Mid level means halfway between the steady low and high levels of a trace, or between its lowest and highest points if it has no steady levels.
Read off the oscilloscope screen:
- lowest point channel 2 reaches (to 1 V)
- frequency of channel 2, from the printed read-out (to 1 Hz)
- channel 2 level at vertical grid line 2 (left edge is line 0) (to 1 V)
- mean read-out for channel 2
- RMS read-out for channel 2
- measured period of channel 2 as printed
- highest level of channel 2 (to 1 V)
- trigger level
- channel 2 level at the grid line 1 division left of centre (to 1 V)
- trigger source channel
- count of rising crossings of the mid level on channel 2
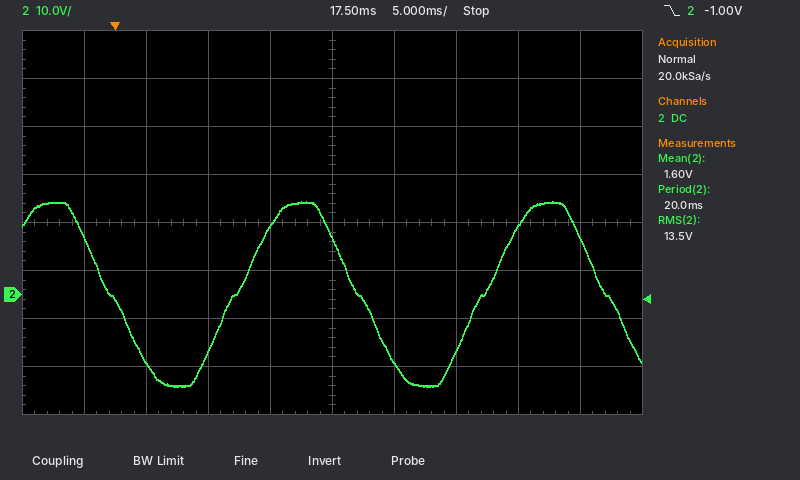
-19 V
50 Hz
-14 V
1.60 V
13.5 V
20.0 ms
19 V
-1.00 V
14 V
channel 2
2
